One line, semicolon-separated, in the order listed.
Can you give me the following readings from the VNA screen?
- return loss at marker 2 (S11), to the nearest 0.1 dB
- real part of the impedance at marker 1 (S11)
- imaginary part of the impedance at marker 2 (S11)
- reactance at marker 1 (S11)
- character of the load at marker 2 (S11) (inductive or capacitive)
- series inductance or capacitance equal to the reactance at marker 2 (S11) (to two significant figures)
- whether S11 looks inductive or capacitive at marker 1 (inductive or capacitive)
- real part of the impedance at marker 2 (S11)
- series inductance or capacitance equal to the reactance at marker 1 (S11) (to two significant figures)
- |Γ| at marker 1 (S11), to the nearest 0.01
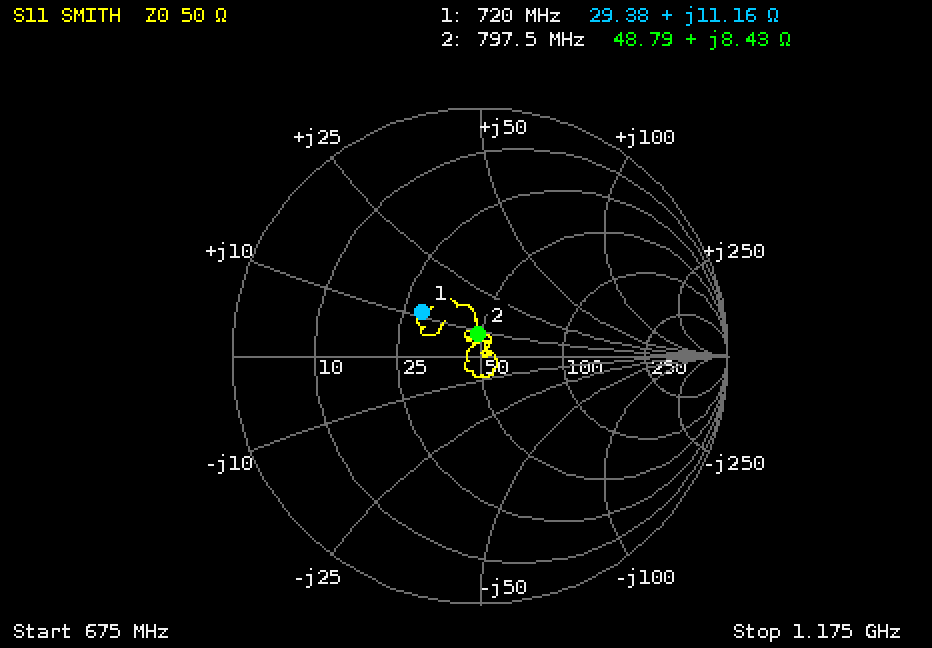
21.3 dB; 29.38 Ω; +8.43 Ω; +11.16 Ω; inductive; 1.7 nH; inductive; 48.79 Ω; 2.5 nH; 0.29
